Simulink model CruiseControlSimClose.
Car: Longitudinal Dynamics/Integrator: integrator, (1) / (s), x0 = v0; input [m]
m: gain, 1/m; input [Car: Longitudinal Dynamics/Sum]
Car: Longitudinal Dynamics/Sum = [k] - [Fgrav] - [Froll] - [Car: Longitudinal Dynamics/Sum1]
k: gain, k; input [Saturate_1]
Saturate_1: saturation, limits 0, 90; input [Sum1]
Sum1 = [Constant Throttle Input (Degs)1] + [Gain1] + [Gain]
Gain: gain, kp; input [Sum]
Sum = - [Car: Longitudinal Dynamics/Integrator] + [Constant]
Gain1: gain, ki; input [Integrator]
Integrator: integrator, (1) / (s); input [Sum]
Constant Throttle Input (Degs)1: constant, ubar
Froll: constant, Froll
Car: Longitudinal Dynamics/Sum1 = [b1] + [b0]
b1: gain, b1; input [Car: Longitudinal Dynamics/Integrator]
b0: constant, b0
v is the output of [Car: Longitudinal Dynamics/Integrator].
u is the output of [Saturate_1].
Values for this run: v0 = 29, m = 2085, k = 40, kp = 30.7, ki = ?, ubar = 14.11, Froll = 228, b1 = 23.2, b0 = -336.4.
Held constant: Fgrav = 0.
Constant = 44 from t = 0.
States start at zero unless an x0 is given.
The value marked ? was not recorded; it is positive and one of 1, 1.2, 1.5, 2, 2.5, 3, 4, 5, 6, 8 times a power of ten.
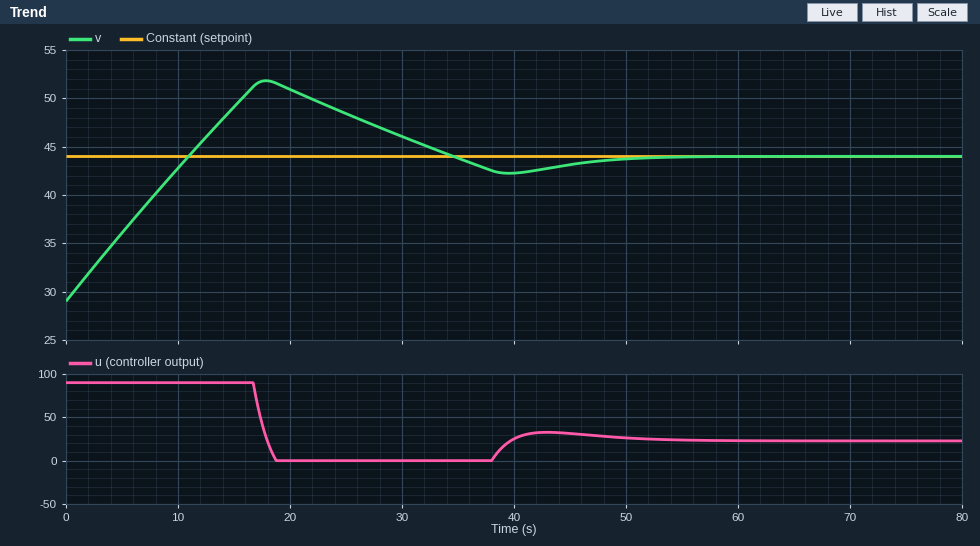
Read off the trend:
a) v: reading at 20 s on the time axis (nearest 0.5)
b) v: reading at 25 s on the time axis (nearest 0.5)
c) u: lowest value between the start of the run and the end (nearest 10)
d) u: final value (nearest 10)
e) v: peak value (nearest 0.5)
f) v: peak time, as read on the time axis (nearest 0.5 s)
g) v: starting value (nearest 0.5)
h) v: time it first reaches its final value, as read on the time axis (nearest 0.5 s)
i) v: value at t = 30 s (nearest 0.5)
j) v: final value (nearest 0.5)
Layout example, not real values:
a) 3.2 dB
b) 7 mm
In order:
a) 51.0
b) 48.5
c) 0
d) 20
e) 52.0
f) 18.0 s
g) 29.0
h) 11.0 s
i) 46.0
j) 44.0
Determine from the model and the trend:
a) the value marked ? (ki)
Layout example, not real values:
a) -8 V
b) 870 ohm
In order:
a) 5
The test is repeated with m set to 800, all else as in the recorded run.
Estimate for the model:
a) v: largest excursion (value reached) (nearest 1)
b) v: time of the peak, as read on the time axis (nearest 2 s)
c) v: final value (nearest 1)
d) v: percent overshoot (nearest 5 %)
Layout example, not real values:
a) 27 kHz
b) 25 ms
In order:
a) 48
b) 6 s
c) 44
d) 25 %
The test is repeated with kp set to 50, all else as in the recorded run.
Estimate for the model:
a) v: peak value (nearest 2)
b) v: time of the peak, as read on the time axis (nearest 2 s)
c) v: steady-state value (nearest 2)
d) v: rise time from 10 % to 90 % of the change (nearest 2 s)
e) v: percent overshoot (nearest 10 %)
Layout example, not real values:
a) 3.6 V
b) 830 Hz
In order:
a) 50
b) 16 s
c) 44
d) 8 s
e) 40 %
